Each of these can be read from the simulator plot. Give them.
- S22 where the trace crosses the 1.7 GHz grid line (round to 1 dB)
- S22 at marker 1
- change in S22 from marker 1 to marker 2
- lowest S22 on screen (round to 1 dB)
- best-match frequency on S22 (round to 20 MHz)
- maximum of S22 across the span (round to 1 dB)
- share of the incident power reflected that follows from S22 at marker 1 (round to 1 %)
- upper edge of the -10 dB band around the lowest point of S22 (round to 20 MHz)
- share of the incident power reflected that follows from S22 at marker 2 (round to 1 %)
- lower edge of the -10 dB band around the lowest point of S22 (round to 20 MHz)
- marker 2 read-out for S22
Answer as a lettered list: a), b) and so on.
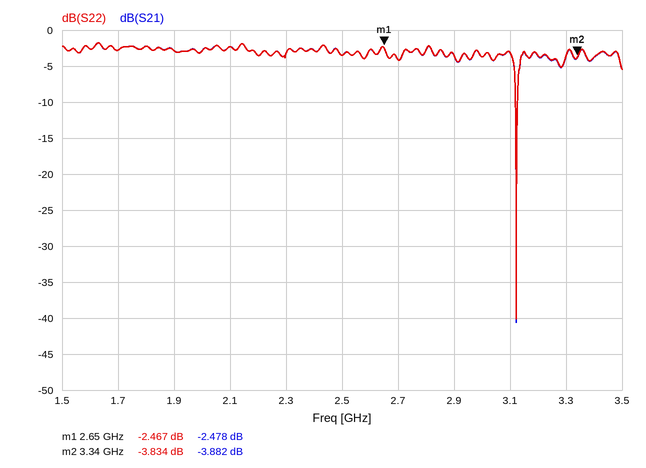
a) -3 dB
b) -2.467 dB
c) -1.367 dB
d) -40 dB
e) 3.12 GHz
f) -2 dB
g) 57 %
h) 3.12 GHz
i) 41 %
j) 3.12 GHz
k) -3.834 dB
